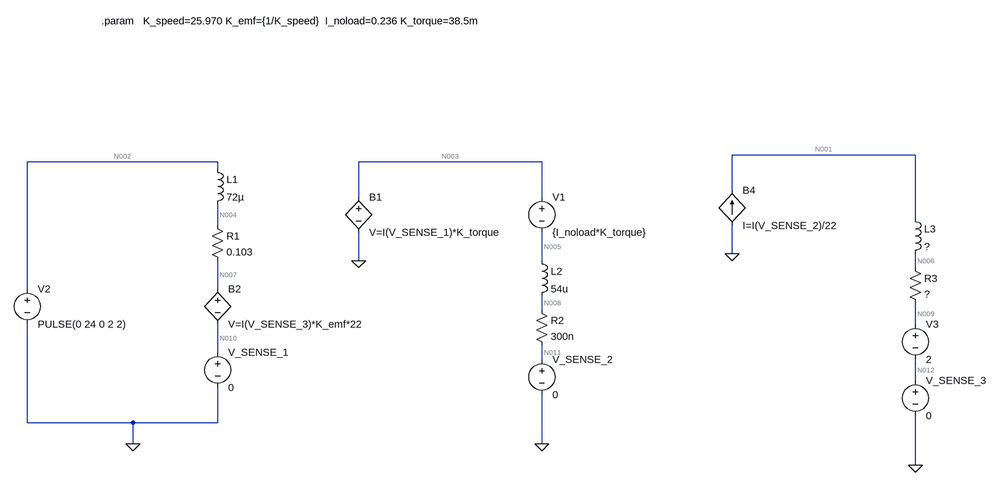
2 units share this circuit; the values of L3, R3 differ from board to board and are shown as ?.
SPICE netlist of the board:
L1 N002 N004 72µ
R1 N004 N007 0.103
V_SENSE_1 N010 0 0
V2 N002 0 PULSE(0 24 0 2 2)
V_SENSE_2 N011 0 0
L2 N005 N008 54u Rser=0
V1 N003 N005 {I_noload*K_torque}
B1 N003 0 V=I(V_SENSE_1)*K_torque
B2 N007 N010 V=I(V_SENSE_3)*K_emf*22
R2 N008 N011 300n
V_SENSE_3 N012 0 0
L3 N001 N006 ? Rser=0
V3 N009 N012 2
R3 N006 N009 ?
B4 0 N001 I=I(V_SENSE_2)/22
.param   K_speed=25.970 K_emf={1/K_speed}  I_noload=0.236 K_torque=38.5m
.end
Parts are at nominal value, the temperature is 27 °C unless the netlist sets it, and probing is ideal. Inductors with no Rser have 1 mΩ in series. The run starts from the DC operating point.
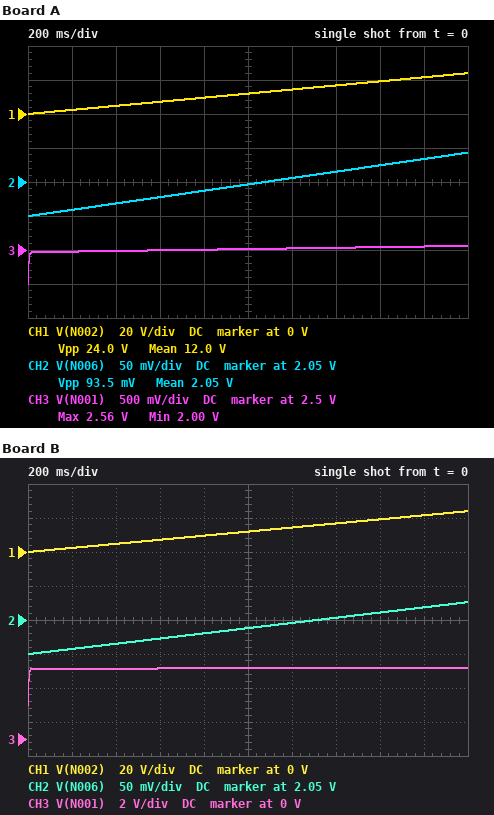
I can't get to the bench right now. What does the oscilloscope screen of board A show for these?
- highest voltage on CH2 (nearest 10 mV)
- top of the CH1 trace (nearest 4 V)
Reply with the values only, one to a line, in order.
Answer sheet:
2.09 V
24 V
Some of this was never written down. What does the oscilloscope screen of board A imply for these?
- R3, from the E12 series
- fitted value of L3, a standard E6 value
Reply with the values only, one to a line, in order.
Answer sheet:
3.3 mΩ
33 mH
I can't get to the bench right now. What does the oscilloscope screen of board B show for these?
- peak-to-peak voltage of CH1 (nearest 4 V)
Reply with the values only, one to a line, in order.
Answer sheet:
24 V
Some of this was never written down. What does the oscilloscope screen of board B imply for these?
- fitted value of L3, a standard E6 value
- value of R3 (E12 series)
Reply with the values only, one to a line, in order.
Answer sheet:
150 mH
2.7 mΩ
